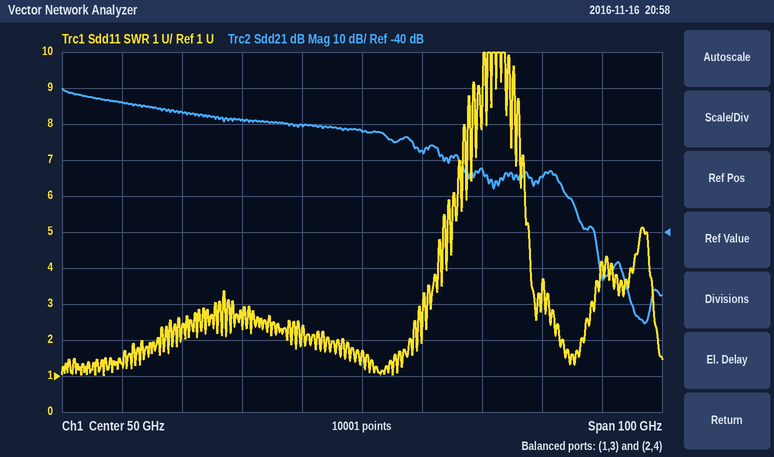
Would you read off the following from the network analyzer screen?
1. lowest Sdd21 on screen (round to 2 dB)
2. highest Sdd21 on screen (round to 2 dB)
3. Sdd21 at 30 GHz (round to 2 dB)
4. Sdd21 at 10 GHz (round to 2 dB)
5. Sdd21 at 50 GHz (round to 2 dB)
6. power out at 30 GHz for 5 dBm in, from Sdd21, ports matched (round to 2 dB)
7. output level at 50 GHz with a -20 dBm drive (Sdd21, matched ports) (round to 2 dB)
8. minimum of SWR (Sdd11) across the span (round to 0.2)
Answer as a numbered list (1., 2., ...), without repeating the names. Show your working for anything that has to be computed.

1. -66 dB
2. 0 dB
3. -8 dB
4. -4 dB
5. -12 dB
6. 5 dBm + (-8 dB) = -4 dBm
7. -20 dBm + (-12 dB) = -32 dBm
8. 1.0
